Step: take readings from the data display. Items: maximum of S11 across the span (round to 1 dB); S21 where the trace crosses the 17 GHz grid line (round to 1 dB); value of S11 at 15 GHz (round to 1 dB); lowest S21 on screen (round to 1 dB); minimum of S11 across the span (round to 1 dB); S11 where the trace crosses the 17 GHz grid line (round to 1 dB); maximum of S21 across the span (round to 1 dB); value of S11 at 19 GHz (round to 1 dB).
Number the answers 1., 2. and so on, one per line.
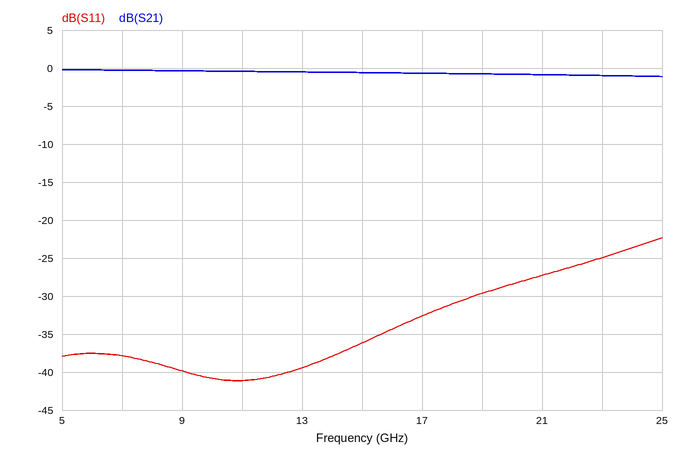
1. -22 dB
2. -1 dB
3. -36 dB
4. -1 dB
5. -41 dB
6. -33 dB
7. 0 dB
8. -30 dB
